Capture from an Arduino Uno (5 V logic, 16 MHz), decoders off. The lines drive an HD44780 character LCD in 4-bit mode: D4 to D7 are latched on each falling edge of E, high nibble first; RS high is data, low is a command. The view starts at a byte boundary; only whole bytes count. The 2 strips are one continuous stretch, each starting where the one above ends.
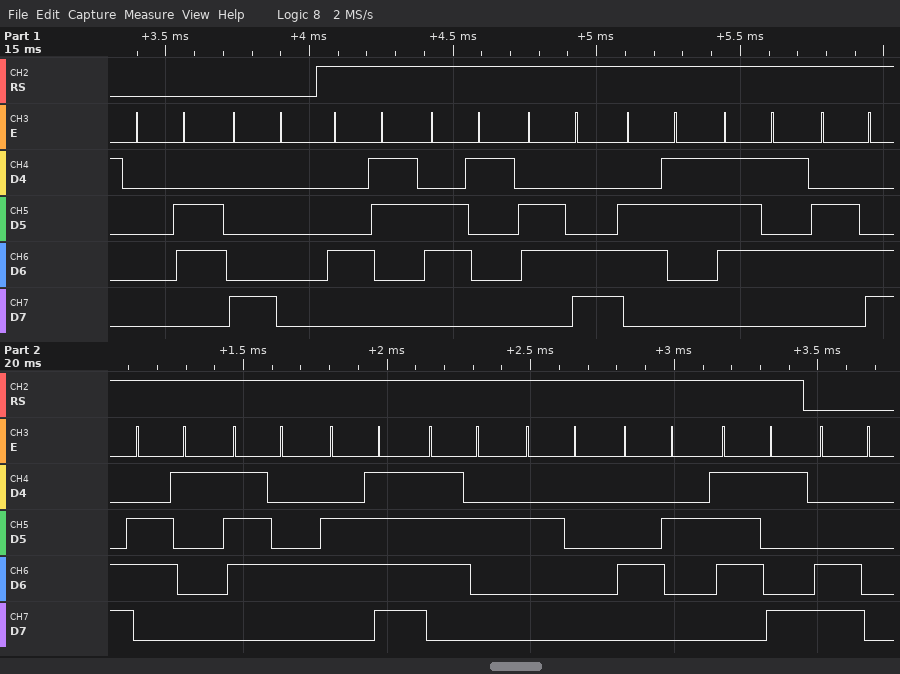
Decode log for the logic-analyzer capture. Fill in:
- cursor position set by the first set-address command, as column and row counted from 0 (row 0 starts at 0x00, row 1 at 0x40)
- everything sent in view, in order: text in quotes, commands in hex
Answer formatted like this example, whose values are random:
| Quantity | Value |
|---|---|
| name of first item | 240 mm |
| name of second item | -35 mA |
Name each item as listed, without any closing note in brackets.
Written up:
| Quantity | Value |
|---|---|
| cursor position set by the first set-address command, as column and row counted from 0 | column 0, row 0 |
| everything sent in view, in order: text in quotes, commands in hex | 0x06 0x80 "Calculator By" 0xC0 |
